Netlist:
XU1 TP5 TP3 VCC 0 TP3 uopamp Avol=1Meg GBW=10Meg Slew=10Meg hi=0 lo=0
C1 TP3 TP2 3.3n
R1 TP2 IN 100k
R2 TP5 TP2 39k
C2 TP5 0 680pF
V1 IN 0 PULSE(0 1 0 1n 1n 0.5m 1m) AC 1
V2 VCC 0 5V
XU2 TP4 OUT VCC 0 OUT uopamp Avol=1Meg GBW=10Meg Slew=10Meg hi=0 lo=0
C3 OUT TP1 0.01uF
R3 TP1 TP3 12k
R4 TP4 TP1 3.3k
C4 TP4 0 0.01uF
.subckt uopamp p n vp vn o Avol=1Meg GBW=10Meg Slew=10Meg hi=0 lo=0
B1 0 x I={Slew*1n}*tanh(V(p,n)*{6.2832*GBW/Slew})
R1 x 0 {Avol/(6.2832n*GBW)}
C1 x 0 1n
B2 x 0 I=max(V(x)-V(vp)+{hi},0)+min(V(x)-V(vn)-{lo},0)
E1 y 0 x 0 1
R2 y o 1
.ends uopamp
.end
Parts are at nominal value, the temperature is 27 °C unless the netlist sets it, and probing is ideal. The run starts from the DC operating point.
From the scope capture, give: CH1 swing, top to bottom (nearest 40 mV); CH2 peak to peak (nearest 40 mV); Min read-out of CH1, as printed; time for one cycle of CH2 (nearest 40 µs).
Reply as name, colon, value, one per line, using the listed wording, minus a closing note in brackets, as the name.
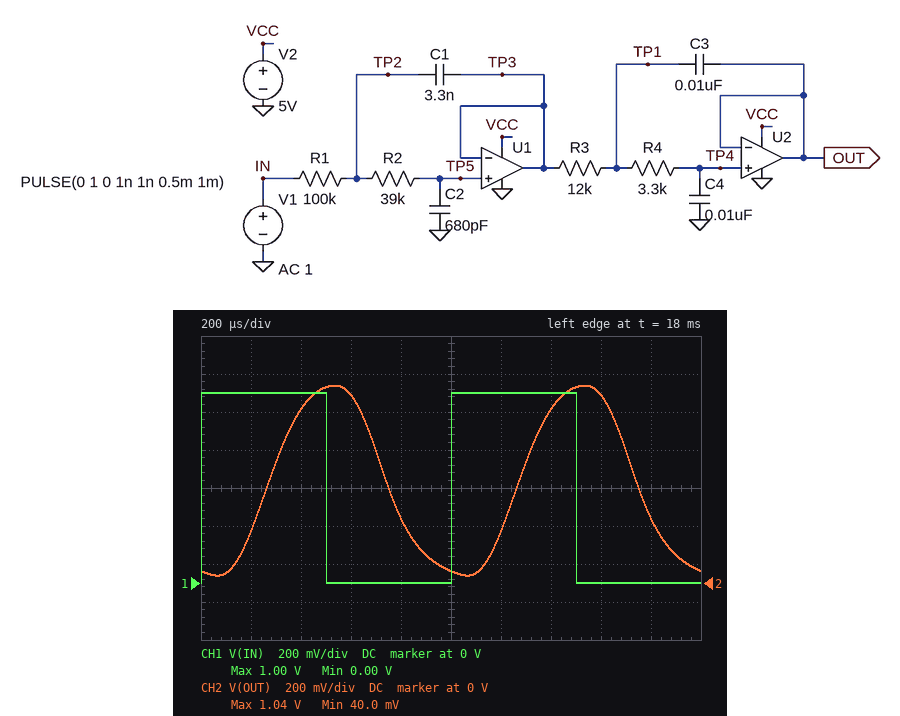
CH1 swing, top to bottom: 1.00 V
CH2 peak to peak: 1.00 V
Min read-out of CH1, as printed: 0.00 V
time for one cycle of CH2: 1.00 ms
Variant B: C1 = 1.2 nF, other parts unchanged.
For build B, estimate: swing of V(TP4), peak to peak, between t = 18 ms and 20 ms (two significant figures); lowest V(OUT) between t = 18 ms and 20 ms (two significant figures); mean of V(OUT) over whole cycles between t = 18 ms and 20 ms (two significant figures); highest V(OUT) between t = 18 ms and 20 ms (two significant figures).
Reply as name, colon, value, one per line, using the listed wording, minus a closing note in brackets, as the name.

swing of V(TP4), peak to peak, between t = 18 ms and 20 ms: 920 mV
lowest V(OUT) between t = 18 ms and 20 ms: 42 mV
mean of V(OUT) over whole cycles between t = 18 ms and 20 ms: 500 mV
highest V(OUT) between t = 18 ms and 20 ms: 960 mV
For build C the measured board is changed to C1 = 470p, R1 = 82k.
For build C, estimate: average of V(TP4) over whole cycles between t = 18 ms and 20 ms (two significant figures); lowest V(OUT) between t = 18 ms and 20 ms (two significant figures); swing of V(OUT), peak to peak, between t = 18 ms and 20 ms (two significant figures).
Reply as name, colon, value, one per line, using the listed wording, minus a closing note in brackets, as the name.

average of V(TP4) over whole cycles between t = 18 ms and 20 ms: 500 mV
lowest V(OUT) between t = 18 ms and 20 ms: 45 mV
swing of V(OUT), peak to peak, between t = 18 ms and 20 ms: 910 mV
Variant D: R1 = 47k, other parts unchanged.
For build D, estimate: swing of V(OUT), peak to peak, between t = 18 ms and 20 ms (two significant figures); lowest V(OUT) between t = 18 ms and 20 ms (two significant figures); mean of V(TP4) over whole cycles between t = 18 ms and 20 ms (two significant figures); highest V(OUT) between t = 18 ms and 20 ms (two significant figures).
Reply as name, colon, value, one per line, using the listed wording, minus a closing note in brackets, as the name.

swing of V(OUT), peak to peak, between t = 18 ms and 20 ms: 960 mV
lowest V(OUT) between t = 18 ms and 20 ms: 31 mV
mean of V(TP4) over whole cycles between t = 18 ms and 20 ms: 520 mV
highest V(OUT) between t = 18 ms and 20 ms: 990 mV
